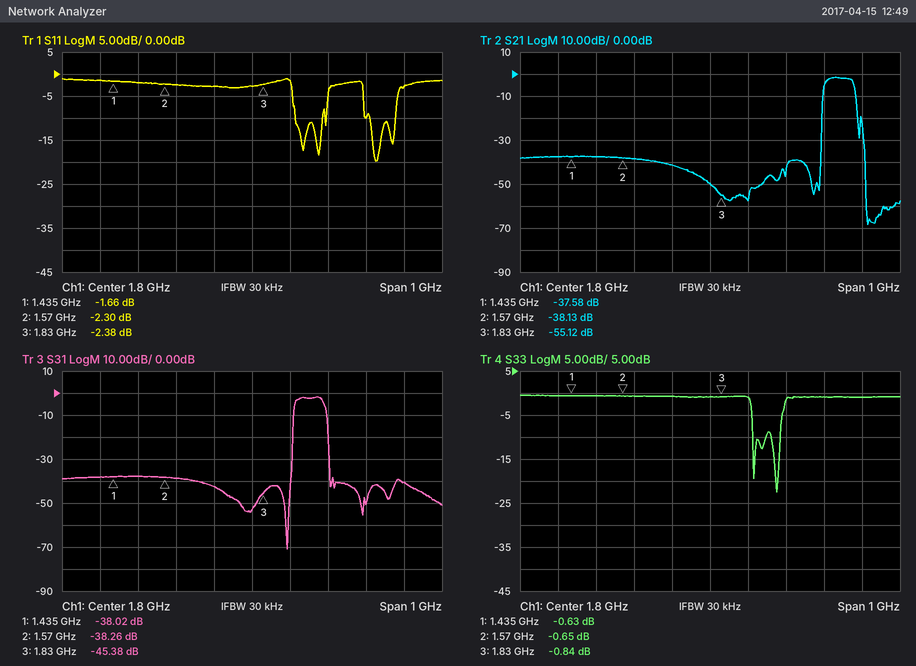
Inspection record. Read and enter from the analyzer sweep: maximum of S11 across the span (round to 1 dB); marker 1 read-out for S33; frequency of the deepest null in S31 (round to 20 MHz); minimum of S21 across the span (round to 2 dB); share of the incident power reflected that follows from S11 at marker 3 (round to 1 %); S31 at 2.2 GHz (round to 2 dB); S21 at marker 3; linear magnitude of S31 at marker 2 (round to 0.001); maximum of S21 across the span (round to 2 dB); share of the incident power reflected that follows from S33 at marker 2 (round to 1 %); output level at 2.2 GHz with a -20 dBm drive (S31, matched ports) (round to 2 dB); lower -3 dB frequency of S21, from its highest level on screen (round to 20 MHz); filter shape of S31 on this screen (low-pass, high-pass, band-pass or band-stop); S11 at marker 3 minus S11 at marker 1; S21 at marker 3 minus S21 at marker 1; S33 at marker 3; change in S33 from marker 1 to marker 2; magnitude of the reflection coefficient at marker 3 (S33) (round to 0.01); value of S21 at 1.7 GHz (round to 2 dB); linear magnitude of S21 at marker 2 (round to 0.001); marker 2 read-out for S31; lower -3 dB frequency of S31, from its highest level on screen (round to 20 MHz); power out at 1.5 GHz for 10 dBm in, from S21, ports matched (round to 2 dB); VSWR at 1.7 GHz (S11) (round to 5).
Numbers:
-1 dB
-0.63 dB
1.90 GHz
-68 dB
58 %
-40 dB
-55.12 dB
0.012
-2 dB
86 %
-60 dBm
2.10 GHz
band-pass
-0.72 dB
-17.54 dB
-0.84 dB
-0.02 dB
0.91
-42 dB
0.012
-38.26 dB
1.92 GHz
-28 dBm
5
